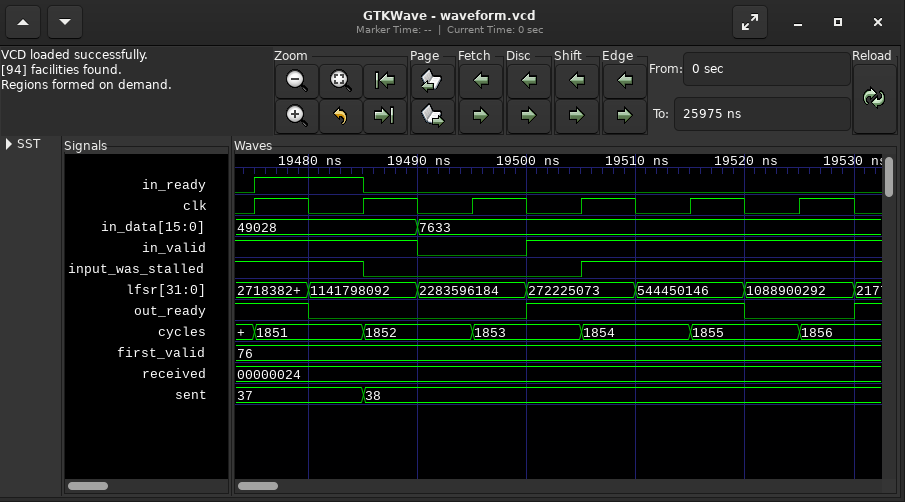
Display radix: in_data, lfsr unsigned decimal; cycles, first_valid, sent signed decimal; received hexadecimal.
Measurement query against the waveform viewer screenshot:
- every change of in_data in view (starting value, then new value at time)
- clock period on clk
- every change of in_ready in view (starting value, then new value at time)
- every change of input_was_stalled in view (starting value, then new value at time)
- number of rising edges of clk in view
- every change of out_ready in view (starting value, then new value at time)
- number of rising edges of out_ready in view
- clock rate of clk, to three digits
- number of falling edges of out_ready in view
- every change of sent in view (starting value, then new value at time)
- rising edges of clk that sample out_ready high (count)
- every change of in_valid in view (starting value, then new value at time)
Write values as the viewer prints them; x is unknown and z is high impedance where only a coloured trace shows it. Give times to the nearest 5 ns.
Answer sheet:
49028, 7633 at 19490 ns
10 ns
0, 1 at 19475 ns, 0 at 19485 ns
1, 0 at 19485 ns, 1 at 19505 ns
6
1, 0 at 19480 ns, 1 at 19500 ns, 0 at 19520 ns, 1 at 19530 ns
2
100 MHz
2
37, 38 at 19485 ns
3
1, 0 at 19490 ns, 1 at 19500 ns
